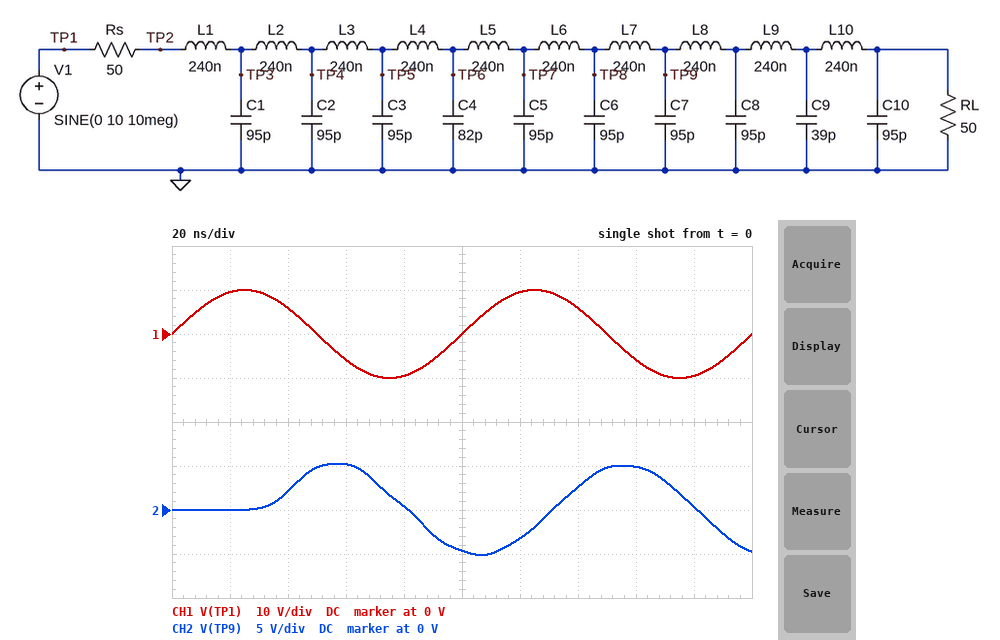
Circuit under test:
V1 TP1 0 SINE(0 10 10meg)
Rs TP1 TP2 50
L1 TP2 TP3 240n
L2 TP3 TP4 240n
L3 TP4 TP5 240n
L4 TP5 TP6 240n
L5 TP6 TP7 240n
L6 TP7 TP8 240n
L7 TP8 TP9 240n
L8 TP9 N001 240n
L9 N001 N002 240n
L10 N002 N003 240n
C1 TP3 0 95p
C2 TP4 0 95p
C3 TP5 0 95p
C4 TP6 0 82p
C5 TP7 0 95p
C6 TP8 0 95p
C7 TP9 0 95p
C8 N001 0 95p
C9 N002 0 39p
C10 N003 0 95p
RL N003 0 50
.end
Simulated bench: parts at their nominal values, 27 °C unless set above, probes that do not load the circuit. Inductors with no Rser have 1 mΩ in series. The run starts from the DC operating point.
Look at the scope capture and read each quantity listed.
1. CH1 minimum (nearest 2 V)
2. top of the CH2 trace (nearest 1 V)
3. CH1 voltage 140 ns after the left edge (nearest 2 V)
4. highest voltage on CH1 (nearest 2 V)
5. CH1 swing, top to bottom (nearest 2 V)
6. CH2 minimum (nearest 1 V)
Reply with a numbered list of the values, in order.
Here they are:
1. -10 V
2. 5 V
3. 6 V
4. 10 V
5. 20 V
6. -5 V
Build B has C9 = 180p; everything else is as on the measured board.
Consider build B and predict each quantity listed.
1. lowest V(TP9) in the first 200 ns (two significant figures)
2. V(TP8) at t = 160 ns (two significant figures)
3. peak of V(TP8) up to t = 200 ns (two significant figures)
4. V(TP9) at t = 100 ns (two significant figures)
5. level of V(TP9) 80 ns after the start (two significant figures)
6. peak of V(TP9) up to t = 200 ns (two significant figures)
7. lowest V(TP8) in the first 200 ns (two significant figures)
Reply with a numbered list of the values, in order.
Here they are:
1. -4.2 V
2. 3.5 V
3. 4.9 V
4. -3.6 V
5. 460 mV
6. 4.7 V
7. -4.3 V
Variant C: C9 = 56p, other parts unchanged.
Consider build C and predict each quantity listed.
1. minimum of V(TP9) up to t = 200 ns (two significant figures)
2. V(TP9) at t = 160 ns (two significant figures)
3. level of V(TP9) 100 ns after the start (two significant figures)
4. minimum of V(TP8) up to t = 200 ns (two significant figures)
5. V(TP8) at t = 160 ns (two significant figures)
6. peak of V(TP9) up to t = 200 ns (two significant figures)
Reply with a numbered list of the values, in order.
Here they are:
1. -5.0 V
2. 4.8 V
3. -4.5 V
4. -5.2 V
5. 4.4 V
6. 5.1 V
